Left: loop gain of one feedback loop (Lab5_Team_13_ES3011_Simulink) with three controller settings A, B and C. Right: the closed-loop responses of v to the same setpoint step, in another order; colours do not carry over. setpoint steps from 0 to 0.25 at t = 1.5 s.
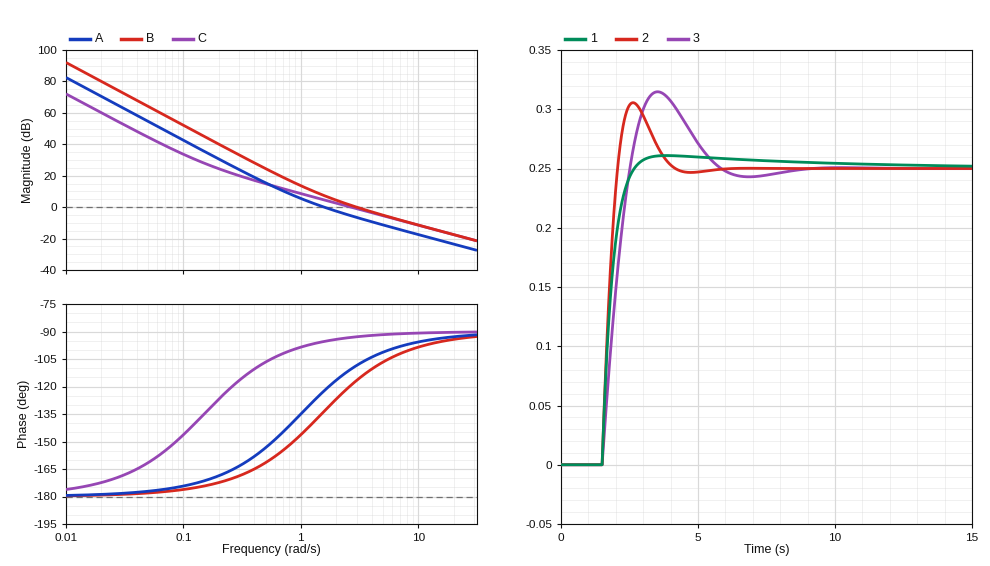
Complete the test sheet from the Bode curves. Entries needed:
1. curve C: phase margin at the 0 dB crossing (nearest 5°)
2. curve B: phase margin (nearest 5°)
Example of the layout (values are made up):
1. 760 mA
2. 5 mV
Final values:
1. 85°
2. 65°
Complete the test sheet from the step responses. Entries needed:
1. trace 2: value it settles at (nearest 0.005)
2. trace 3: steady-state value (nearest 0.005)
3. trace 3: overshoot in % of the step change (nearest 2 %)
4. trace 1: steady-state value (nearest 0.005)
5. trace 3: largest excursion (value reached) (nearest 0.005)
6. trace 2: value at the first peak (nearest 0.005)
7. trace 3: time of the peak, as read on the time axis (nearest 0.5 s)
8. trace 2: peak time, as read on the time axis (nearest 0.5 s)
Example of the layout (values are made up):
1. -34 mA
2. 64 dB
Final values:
1. 0.250
2. 0.250
3. 26 %
4. 0.250
5. 0.315
6. 0.305
7. 3.5 s
8. 2.5 s
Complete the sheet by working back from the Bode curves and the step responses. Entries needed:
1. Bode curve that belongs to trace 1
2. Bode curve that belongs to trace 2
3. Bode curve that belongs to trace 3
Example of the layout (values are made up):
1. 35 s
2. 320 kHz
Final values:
1. C
2. B
3. A
